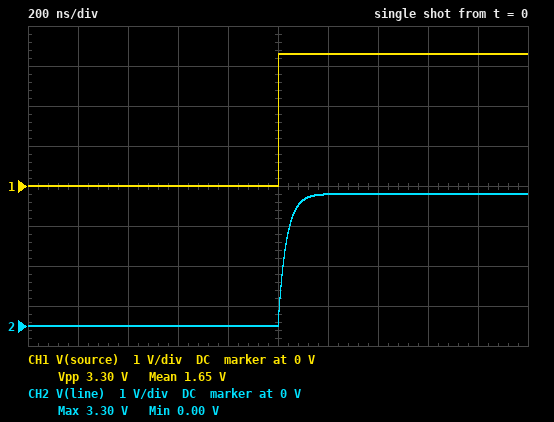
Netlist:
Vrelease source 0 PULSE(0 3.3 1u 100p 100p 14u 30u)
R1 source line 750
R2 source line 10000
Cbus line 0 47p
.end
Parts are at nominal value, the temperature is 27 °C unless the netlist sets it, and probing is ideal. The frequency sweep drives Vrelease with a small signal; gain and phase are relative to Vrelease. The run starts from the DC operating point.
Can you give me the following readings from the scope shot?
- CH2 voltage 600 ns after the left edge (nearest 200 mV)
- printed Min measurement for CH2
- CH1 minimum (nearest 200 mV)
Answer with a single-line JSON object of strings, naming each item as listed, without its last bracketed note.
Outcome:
{"CH2 voltage 600 ns after the left edge": "0 V", "printed Min measurement for CH2": "0.00 V", "CH1 minimum": "0 V"}
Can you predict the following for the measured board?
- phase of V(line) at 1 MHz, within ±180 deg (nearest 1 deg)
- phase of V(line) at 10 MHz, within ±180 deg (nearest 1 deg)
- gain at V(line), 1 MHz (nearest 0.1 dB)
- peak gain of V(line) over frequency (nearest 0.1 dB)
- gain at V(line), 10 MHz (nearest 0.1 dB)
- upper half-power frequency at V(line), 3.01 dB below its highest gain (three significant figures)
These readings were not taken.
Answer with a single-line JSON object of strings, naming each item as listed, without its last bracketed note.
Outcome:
{"phase of V(line) at 1 MHz, within ±180 deg": "-12 deg", "phase of V(line) at 10 MHz, within ±180 deg": "-64 deg", "gain at V(line), 1 MHz": "-0.2 dB", "peak gain of V(line) over frequency": "0 dB", "gain at V(line), 10 MHz": "-7.2 dB", "upper half-power frequency at V(line), 3.01 dB below its highest gain": "4.85 MHz"}
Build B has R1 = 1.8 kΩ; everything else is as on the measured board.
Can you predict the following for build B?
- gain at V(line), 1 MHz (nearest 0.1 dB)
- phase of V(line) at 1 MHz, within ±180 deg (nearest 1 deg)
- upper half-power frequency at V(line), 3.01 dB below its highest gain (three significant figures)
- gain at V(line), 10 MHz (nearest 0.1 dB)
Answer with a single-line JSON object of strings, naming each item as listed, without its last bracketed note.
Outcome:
{"gain at V(line), 1 MHz": "-0.8 dB", "phase of V(line) at 1 MHz, within ±180 deg": "-24 deg", "upper half-power frequency at V(line), 3.01 dB below its highest gain": "2.22 MHz", "gain at V(line), 10 MHz": "-13.3 dB"}
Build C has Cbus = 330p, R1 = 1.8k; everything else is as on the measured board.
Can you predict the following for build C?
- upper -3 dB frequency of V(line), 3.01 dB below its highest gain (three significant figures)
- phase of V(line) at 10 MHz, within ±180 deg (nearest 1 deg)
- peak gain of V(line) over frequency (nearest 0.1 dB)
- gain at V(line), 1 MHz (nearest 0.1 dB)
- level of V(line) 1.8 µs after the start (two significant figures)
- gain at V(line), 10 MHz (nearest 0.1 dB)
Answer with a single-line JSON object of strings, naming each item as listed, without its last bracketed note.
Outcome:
{"upper -3 dB frequency of V(line), 3.01 dB below its highest gain": "316 kHz", "phase of V(line) at 10 MHz, within ±180 deg": "-88 deg", "peak gain of V(line) over frequency": "0 dB", "gain at V(line), 1 MHz": "-10.4 dB", "level of V(line) 1.8 µs after the start": "2.6 V", "gain at V(line), 10 MHz": "-30.0 dB"}
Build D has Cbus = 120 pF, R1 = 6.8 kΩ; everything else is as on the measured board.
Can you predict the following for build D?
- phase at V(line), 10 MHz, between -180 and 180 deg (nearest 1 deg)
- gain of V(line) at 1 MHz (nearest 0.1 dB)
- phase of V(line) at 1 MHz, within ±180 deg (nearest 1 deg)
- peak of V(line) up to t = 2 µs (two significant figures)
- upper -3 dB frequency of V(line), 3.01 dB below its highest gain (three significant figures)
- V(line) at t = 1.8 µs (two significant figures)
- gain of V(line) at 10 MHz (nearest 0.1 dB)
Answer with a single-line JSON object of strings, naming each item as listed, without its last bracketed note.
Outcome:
{"phase at V(line), 10 MHz, between -180 and 180 deg": "-88 deg", "gain of V(line) at 1 MHz": "-10.1 dB", "phase of V(line) at 1 MHz, within ±180 deg": "-72 deg", "peak of V(line) up to t = 2 µs": "2.9 V", "upper -3 dB frequency of V(line), 3.01 dB below its highest gain": "328 kHz", "V(line) at t = 1.8 µs": "2.7 V", "gain of V(line) at 10 MHz": "-29.7 dB"}
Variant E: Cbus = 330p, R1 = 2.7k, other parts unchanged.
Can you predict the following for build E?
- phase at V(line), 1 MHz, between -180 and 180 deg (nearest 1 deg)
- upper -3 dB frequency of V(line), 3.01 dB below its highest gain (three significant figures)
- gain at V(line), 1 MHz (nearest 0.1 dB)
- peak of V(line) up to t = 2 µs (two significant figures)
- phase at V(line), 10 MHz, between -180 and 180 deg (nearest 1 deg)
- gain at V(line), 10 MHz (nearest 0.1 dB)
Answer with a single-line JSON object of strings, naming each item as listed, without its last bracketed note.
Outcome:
{"phase at V(line), 1 MHz, between -180 and 180 deg": "-77 deg", "upper -3 dB frequency of V(line), 3.01 dB below its highest gain": "227 kHz", "gain at V(line), 1 MHz": "-13.1 dB", "peak of V(line) up to t = 2 µs": "2.5 V", "phase at V(line), 10 MHz, between -180 and 180 deg": "-89 deg", "gain at V(line), 10 MHz": "-32.9 dB"}
